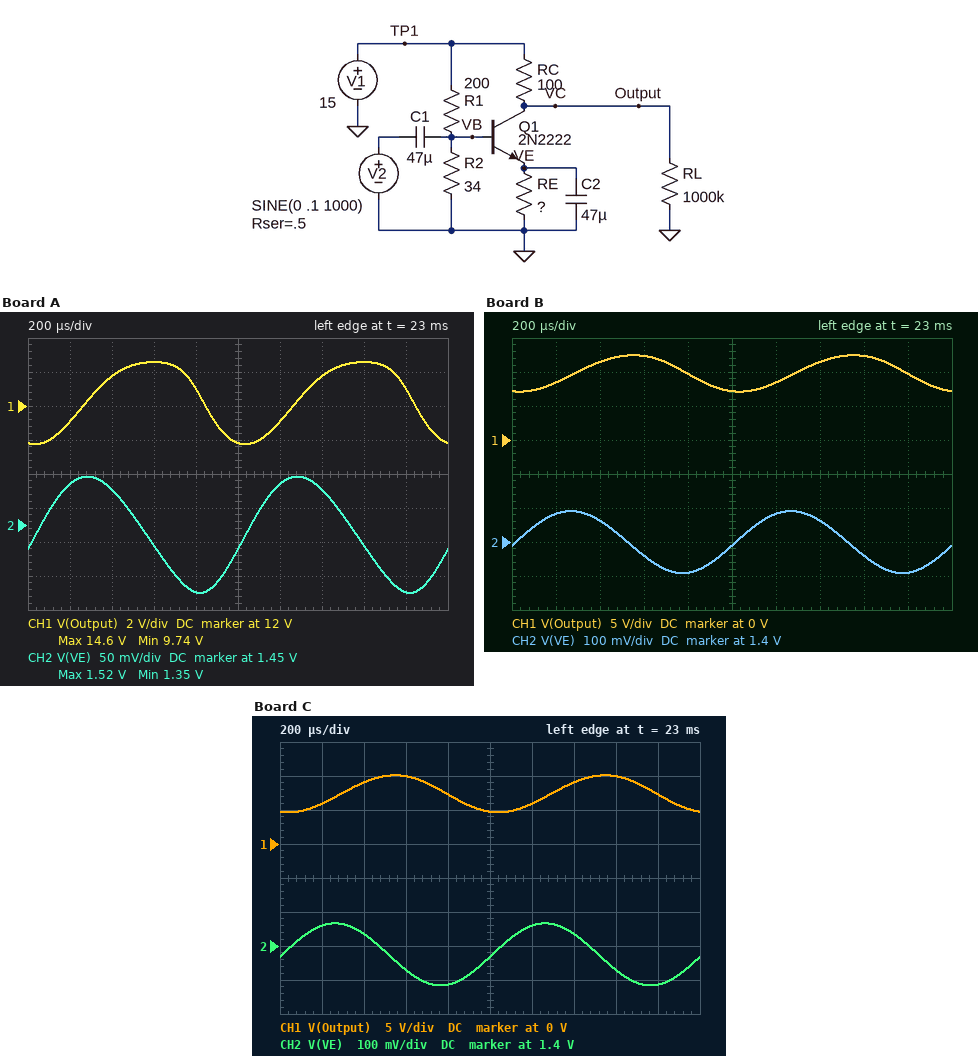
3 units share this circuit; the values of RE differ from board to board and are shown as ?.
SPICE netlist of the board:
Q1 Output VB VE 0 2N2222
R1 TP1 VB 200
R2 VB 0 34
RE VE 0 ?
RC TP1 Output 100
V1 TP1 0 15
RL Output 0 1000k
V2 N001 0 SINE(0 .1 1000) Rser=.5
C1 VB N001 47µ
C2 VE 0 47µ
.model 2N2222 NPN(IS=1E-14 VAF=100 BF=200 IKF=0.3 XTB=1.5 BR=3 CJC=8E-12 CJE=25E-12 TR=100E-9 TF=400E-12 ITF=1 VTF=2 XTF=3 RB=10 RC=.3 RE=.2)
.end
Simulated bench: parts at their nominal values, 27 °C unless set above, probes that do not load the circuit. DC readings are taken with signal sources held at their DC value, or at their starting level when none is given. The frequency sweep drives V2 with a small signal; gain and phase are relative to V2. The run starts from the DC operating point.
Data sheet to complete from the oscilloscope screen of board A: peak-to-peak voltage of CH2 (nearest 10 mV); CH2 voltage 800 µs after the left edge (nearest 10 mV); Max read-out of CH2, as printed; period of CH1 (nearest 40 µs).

170 mV
1.35 V
1.52 V
1.00 ms
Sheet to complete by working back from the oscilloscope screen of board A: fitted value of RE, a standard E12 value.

56 Ω
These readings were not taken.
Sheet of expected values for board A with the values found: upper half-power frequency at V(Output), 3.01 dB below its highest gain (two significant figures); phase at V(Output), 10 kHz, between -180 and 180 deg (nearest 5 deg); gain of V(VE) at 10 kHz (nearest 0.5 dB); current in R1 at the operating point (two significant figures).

26 MHz
-165 deg
-12.5 dB
64 mA
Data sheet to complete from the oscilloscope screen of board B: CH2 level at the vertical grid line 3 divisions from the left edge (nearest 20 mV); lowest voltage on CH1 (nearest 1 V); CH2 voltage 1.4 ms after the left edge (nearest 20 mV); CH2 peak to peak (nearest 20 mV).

1.36 V
7 V
1.46 V
180 mV
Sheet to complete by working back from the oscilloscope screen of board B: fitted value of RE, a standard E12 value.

27 Ω
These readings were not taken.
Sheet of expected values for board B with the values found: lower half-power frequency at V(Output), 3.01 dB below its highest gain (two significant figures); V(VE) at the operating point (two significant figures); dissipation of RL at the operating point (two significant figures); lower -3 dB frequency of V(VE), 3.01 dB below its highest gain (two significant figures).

4.1 kHz
1.4 V
97 µW
110 Hz
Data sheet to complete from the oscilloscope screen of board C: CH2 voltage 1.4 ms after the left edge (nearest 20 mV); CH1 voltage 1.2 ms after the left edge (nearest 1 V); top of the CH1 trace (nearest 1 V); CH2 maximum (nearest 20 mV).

1.44 V
6 V
10 V
1.46 V
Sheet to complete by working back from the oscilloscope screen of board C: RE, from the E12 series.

18 Ω
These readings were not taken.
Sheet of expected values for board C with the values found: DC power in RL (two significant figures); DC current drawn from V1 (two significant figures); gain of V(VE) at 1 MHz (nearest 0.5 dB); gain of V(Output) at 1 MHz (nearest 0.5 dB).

55 µW
140 mA
-46.5 dB
42.5 dB
